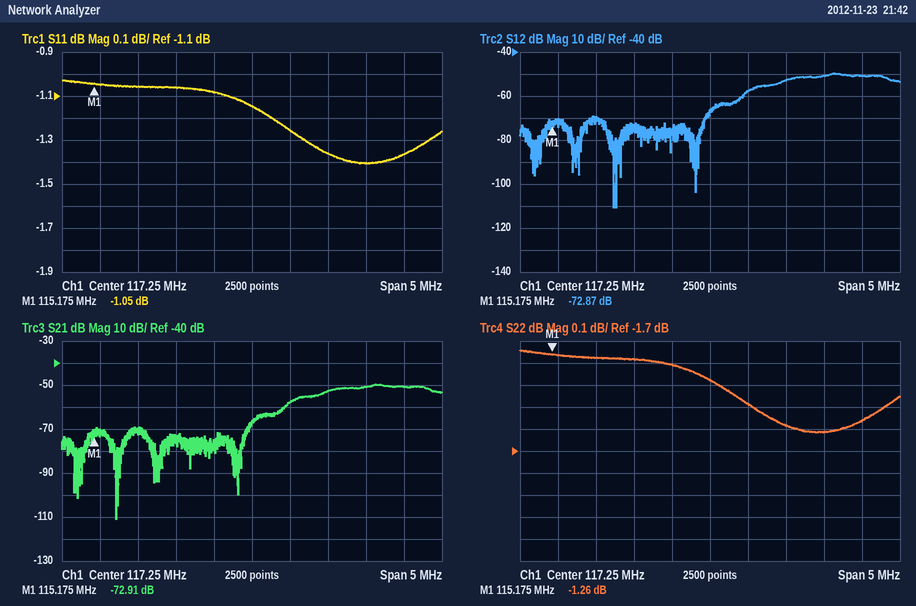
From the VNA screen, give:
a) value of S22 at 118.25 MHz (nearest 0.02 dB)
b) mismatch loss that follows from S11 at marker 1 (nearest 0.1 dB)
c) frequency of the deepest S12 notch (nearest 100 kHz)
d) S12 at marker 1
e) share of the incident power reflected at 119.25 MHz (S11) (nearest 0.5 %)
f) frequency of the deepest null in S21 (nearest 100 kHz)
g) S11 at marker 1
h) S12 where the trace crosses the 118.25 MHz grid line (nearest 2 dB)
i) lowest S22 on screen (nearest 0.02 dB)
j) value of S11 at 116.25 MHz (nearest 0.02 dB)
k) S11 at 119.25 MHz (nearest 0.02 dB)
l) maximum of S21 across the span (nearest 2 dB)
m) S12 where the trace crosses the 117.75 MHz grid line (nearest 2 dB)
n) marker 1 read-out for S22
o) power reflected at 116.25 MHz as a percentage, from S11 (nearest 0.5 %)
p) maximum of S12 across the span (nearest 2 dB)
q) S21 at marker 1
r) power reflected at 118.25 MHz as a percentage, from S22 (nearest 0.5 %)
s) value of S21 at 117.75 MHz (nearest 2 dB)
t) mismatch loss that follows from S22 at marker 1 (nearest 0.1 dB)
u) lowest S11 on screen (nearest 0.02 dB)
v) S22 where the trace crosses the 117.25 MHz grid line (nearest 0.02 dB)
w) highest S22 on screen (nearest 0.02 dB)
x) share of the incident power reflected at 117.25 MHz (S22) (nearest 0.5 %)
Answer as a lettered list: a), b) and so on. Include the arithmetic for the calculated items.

a) -1.58 dB
b) −10 log10(1 − 10^(-1.05/10)) ≈ 6.7 dB
c) 116.0 MHz
d) -72.87 dB
e) 10^(-1.36/10) ≈ 73.1 %, so 73.0 % to the nearest 0.5 %
f) 115.5 MHz
g) -1.05 dB
h) -52 dB
i) -1.62 dB
j) -1.06 dB
k) -1.36 dB
l) -50 dB
m) -58 dB
n) -1.26 dB
o) 10^(-1.06/10) ≈ 78.3 %, so 78.5 % to the nearest 0.5 %
p) -50 dB
q) -72.91 dB
r) 10^(-1.58/10) ≈ 69.5 %
s) -58 dB
t) −10 log10(1 − 10^(-1.26/10)) ≈ 6.0 dB
u) -1.40 dB
v) -1.38 dB
w) -1.24 dB
x) 10^(-1.38/10) ≈ 72.8 %, so 73.0 % to the nearest 0.5 %
